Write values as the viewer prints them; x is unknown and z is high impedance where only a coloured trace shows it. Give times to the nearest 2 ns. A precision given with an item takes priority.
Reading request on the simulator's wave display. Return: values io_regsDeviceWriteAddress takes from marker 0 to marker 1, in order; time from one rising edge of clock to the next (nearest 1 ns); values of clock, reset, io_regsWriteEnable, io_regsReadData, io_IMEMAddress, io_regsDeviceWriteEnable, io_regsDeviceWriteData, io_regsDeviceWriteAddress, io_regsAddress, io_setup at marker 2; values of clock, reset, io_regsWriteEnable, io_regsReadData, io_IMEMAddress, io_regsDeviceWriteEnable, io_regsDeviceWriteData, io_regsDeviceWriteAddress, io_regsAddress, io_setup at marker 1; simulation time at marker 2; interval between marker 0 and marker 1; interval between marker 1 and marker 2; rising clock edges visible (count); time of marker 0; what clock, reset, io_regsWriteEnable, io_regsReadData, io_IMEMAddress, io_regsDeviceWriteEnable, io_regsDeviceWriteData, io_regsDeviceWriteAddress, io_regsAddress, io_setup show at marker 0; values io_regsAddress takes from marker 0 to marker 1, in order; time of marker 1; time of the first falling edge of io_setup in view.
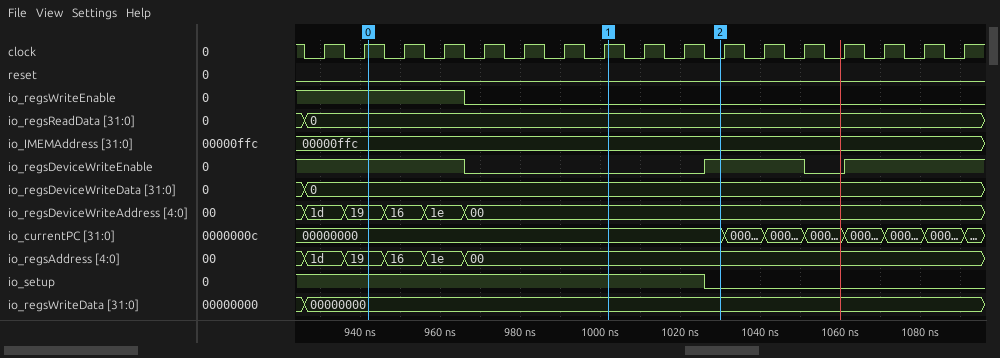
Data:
19, 16, 1e, 00
10 ns
clock=0, reset=0, io_regsWriteEnable=0, io_regsReadData=0, io_IMEMAddress=00000ffc, io_regsDeviceWriteEnable=1, io_regsDeviceWriteData=0, io_regsDeviceWriteAddress=00, io_regsAddress=00, io_setup=0
clock=1, reset=0, io_regsWriteEnable=0, io_regsReadData=0, io_IMEMAddress=00000ffc, io_regsDeviceWriteEnable=0, io_regsDeviceWriteData=0, io_regsDeviceWriteAddress=00, io_regsAddress=00, io_setup=1
1030 ns
60 ns
28 ns
17
942 ns
clock=1, reset=0, io_regsWriteEnable=1, io_regsReadData=0, io_IMEMAddress=00000ffc, io_regsDeviceWriteEnable=1, io_regsDeviceWriteData=0, io_regsDeviceWriteAddress=19, io_regsAddress=19, io_setup=1
19, 16, 1e, 00
1002 ns
1026 ns
